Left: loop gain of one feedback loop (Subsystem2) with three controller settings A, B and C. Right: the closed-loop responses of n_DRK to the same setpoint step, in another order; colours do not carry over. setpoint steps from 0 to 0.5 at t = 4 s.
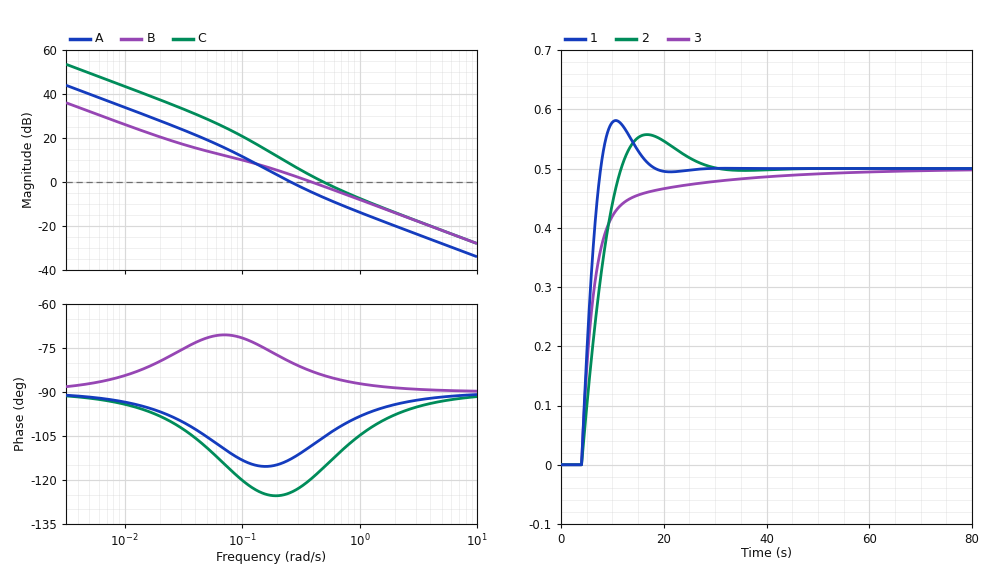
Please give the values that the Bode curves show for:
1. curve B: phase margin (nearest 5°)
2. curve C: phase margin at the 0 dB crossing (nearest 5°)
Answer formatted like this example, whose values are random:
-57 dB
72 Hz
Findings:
95°
65°
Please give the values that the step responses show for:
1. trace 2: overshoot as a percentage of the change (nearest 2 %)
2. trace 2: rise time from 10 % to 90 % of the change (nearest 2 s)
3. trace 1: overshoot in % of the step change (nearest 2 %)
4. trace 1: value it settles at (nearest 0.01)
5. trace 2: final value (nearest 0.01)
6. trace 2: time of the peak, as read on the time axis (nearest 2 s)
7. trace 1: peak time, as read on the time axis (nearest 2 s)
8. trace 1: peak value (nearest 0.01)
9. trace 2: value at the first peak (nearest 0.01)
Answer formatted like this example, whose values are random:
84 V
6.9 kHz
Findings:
12 %
6 s
16 %
0.50
0.50
16 s
10 s
0.58
0.56
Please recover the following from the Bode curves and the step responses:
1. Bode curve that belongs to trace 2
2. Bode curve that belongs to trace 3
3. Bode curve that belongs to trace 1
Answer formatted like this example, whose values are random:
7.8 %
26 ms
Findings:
A
B
C
